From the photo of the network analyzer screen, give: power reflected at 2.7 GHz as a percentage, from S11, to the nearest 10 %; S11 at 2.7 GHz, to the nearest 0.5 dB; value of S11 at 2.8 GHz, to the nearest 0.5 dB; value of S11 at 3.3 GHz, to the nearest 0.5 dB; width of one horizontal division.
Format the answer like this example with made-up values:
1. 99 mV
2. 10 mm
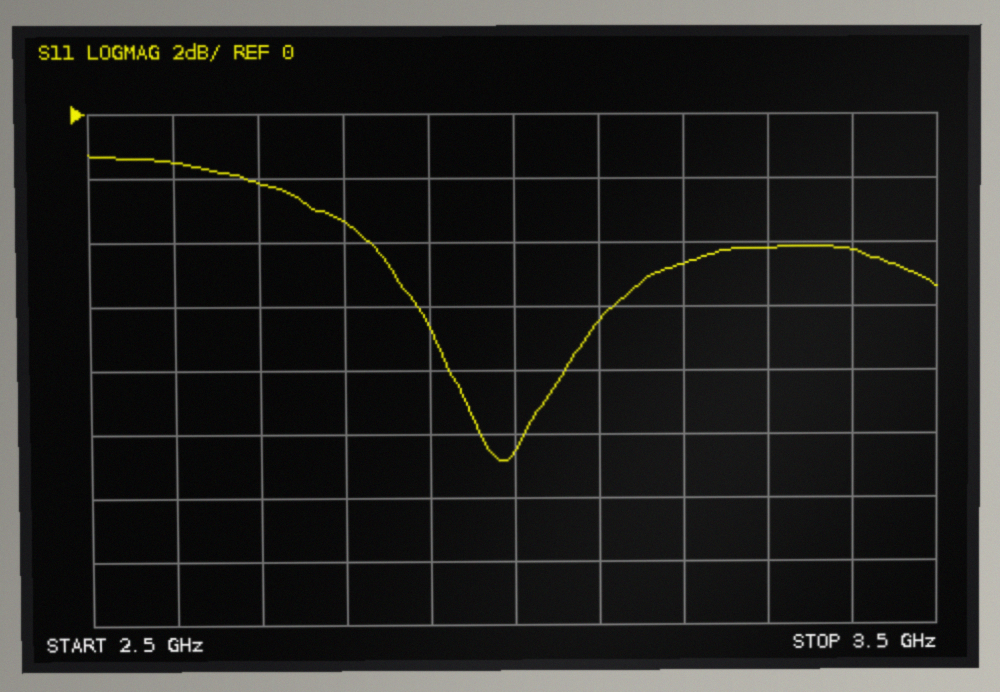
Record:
1. 60 %
2. -2.0 dB
3. -3.5 dB
4. -4.0 dB
5. 100 MHz
